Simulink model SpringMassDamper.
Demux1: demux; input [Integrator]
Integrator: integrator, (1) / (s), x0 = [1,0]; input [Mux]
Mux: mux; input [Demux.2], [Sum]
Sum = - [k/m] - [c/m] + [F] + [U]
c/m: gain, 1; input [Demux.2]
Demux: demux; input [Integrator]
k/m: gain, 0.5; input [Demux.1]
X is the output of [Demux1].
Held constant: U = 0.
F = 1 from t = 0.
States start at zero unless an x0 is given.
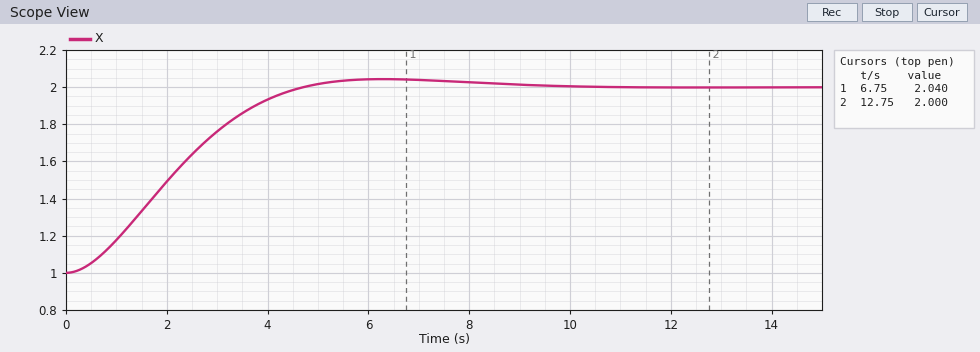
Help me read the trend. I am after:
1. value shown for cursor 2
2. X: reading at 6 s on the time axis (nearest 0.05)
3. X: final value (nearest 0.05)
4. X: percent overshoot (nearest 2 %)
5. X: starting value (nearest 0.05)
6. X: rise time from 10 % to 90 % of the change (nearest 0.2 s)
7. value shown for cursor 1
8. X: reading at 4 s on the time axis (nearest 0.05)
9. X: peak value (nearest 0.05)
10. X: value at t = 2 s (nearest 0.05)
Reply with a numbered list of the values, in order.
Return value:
1. 2.000
2. 2.05
3. 2.00
4. 4 %
5. 1.00
6. 3.0 s
7. 2.040
8. 1.95
9. 2.05
10. 1.50
